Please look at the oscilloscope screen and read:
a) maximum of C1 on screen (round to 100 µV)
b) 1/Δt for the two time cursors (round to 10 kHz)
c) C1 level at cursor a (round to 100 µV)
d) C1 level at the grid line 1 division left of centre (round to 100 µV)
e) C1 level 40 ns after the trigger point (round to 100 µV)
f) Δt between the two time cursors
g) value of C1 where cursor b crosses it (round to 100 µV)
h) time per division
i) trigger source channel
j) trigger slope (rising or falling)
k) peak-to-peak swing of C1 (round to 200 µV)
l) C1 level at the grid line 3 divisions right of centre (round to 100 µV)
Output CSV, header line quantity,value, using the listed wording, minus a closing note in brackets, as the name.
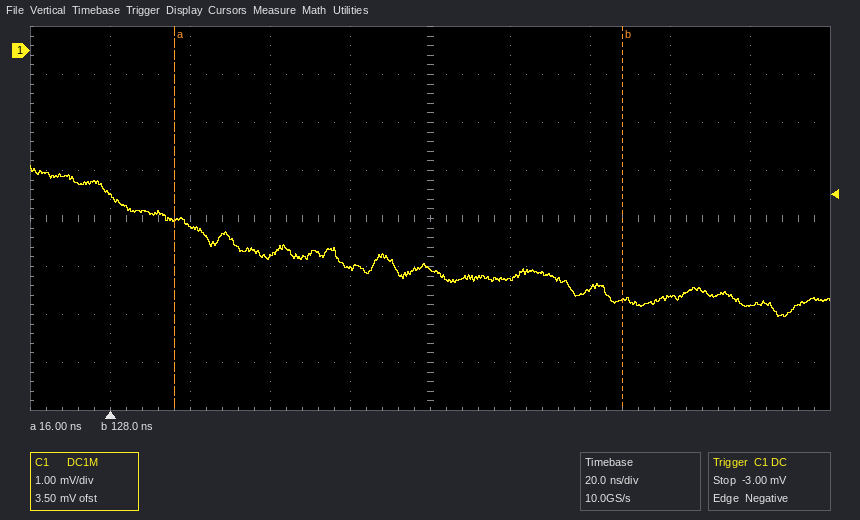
quantity,value
maximum of C1 on screen,-2.4 mV
1/Δt for the two time cursors,8.93 MHz
C1 level at cursor a,-3.5 mV
C1 level at the grid line 1 division left of centre,-4.5 mV
C1 level 40 ns after the trigger point,-4.3 mV
Δt between the two time cursors,112 ns
value of C1 where cursor b crosses it,-5.2 mV
time per division,20 ns
trigger source channel,C1
trigger slope,falling
peak-to-peak swing of C1,3.2 mV
C1 level at the grid line 3 divisions right of centre,-5.1 mV
